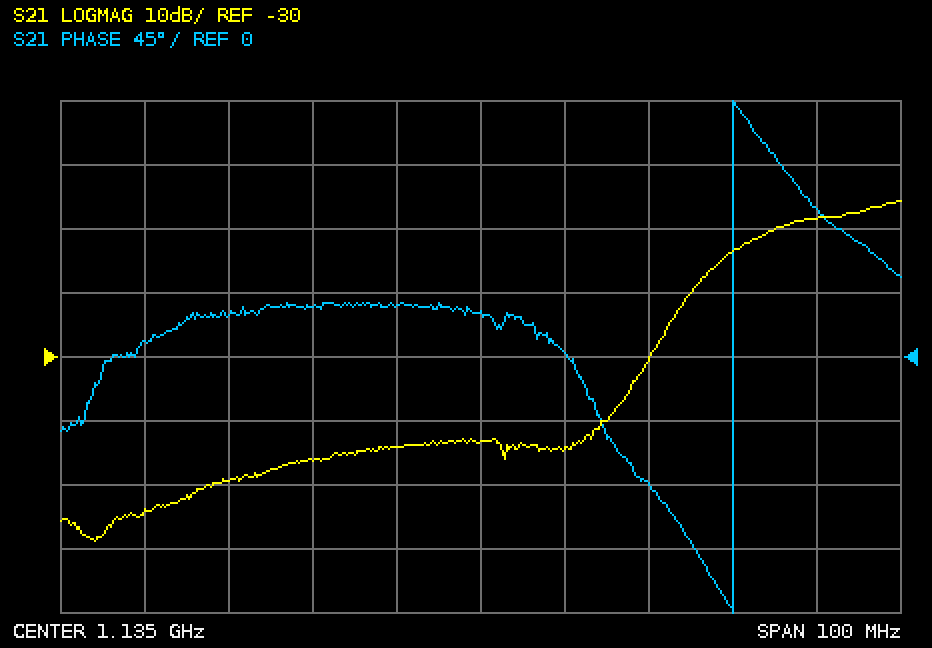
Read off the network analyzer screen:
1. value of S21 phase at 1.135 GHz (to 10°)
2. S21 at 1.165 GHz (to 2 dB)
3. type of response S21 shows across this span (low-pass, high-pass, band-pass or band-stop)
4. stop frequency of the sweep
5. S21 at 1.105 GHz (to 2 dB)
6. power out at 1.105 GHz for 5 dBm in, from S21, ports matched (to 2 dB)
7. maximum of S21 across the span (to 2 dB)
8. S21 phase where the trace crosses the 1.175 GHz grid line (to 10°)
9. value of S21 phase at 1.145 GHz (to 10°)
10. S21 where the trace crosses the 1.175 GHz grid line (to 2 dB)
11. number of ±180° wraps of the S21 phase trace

30°
-14 dB
high-pass
1.185 GHz
-50 dB
-44 dBm
-6 dB
100°
0°
-8 dB
1
